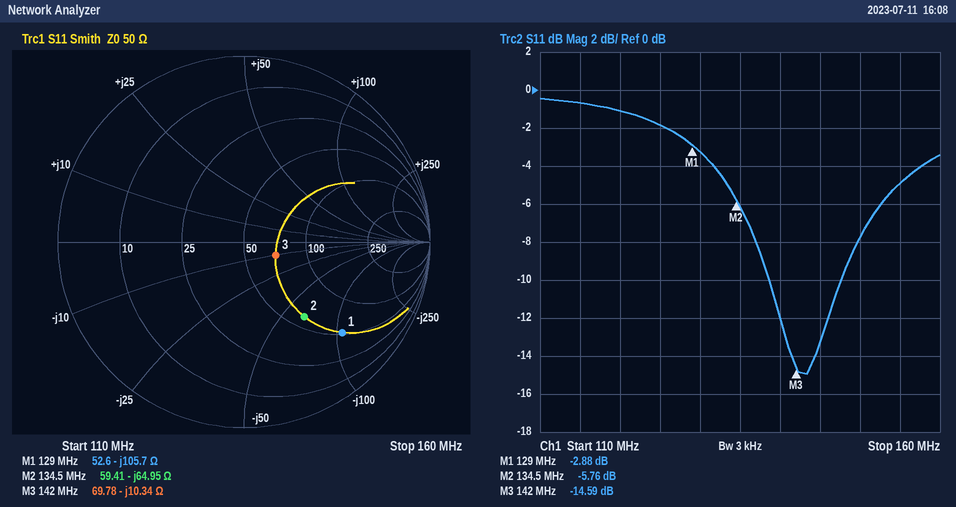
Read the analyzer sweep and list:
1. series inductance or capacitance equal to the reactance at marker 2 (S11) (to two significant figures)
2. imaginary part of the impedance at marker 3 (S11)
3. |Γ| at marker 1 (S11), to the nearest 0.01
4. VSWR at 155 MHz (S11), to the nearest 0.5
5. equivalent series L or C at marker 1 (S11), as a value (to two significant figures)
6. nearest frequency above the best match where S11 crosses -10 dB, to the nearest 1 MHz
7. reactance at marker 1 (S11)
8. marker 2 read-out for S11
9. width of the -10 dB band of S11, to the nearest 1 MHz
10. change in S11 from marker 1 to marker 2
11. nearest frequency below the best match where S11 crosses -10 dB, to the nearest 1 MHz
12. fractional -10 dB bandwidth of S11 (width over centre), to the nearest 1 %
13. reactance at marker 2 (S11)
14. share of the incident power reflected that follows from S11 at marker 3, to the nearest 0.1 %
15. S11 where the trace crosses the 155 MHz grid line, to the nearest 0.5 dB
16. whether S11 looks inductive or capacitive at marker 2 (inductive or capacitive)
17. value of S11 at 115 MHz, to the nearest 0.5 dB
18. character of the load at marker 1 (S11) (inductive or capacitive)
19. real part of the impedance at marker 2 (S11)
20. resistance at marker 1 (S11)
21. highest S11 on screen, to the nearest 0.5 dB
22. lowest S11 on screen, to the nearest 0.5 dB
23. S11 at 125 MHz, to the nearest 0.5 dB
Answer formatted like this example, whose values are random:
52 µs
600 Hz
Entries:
18 pF
-10.34 Ω
0.72
3.5
12 pF
148 MHz
-105.7 Ω
-5.76 dB
9 MHz
-2.88 dB
139 MHz
6 %
-64.95 Ω
3.5 %
-5.0 dB
capacitive
-0.5 dB
capacitive
59.41 Ω
52.6 Ω
-0.5 dB
-15.0 dB
-2.0 dB
